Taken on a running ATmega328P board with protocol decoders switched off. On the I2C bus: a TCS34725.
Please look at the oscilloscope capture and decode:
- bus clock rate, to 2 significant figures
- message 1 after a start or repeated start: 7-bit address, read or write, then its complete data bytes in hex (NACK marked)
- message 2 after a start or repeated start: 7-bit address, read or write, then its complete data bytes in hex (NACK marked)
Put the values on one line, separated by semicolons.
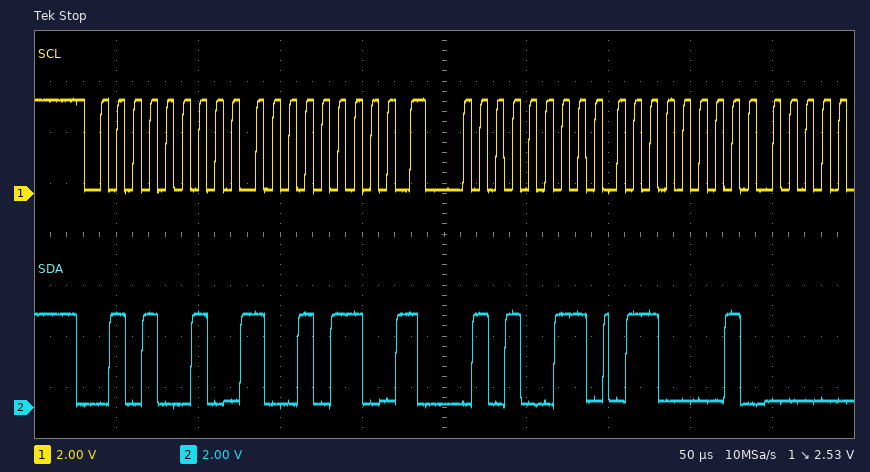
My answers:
100 kHz; 0x29 write: 96; 0x29 read: 61
